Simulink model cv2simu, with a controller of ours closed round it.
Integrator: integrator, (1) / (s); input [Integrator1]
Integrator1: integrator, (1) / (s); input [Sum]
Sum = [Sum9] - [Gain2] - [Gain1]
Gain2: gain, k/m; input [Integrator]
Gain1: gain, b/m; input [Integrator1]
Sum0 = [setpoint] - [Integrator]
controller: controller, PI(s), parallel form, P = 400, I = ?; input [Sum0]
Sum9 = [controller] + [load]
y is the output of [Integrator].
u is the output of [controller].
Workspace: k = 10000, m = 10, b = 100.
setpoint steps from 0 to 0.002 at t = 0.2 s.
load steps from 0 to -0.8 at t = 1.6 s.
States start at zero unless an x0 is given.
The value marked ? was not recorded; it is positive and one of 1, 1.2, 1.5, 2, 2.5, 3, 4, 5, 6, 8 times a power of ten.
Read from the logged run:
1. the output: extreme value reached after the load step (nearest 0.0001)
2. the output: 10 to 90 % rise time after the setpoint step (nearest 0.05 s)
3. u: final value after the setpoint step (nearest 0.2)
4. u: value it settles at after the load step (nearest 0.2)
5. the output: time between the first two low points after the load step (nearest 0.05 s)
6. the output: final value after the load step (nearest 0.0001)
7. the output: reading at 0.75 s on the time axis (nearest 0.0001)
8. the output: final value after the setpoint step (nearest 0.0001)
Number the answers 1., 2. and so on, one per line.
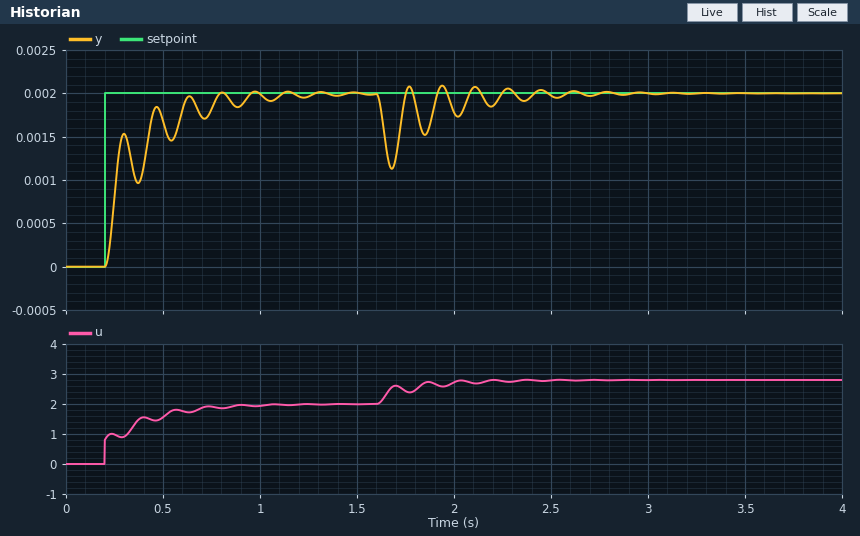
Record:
1. 0.0011
2. 0.25 s
3. 2.0
4. 2.8
5. 0.15 s
6. 0.0020
7. 0.0018
8. 0.0020
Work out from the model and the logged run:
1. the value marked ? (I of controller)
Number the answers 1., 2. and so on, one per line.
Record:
1. 6000
